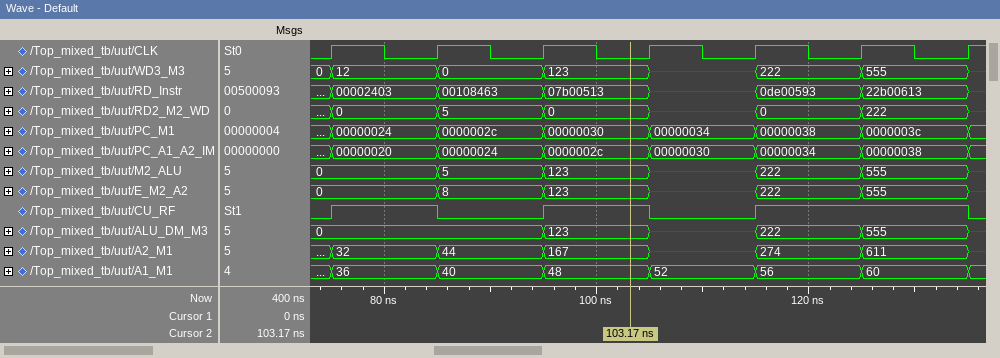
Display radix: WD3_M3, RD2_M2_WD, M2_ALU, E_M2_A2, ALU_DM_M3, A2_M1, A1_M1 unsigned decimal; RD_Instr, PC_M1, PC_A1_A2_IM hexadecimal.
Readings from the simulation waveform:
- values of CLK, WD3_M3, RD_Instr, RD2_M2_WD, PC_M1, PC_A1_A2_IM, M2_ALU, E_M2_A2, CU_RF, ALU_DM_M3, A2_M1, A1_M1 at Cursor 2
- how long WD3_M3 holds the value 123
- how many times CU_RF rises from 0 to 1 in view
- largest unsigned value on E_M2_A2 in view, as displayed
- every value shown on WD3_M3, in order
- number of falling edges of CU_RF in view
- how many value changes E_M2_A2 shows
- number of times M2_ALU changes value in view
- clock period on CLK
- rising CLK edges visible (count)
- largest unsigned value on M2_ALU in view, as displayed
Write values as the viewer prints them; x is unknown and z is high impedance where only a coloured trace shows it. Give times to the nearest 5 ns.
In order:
CLK=0, WD3_M3=123, RD_Instr=07b00513, RD2_M2_WD=0, PC_M1=00000030, PC_A1_A2_IM=0000002c, M2_ALU=123, E_M2_A2=123, CU_RF=1, ALU_DM_M3=123, A2_M1=167, A1_M1=48
10 ns
3
555
0, 12, 0, 123, x, 222, 555, x
3
6
6
10 ns
7
555
